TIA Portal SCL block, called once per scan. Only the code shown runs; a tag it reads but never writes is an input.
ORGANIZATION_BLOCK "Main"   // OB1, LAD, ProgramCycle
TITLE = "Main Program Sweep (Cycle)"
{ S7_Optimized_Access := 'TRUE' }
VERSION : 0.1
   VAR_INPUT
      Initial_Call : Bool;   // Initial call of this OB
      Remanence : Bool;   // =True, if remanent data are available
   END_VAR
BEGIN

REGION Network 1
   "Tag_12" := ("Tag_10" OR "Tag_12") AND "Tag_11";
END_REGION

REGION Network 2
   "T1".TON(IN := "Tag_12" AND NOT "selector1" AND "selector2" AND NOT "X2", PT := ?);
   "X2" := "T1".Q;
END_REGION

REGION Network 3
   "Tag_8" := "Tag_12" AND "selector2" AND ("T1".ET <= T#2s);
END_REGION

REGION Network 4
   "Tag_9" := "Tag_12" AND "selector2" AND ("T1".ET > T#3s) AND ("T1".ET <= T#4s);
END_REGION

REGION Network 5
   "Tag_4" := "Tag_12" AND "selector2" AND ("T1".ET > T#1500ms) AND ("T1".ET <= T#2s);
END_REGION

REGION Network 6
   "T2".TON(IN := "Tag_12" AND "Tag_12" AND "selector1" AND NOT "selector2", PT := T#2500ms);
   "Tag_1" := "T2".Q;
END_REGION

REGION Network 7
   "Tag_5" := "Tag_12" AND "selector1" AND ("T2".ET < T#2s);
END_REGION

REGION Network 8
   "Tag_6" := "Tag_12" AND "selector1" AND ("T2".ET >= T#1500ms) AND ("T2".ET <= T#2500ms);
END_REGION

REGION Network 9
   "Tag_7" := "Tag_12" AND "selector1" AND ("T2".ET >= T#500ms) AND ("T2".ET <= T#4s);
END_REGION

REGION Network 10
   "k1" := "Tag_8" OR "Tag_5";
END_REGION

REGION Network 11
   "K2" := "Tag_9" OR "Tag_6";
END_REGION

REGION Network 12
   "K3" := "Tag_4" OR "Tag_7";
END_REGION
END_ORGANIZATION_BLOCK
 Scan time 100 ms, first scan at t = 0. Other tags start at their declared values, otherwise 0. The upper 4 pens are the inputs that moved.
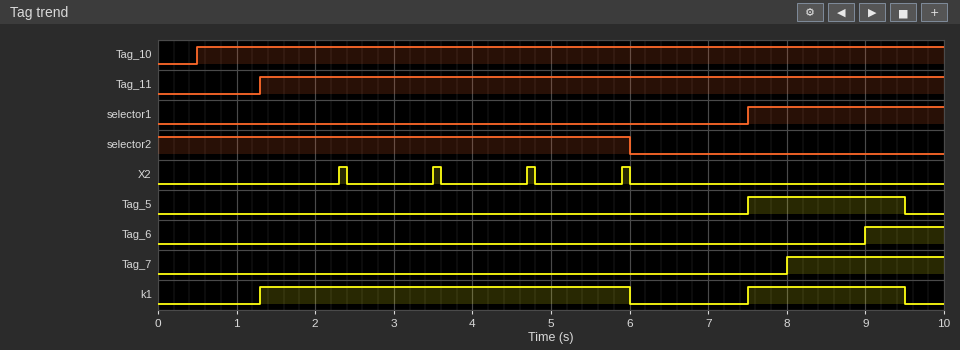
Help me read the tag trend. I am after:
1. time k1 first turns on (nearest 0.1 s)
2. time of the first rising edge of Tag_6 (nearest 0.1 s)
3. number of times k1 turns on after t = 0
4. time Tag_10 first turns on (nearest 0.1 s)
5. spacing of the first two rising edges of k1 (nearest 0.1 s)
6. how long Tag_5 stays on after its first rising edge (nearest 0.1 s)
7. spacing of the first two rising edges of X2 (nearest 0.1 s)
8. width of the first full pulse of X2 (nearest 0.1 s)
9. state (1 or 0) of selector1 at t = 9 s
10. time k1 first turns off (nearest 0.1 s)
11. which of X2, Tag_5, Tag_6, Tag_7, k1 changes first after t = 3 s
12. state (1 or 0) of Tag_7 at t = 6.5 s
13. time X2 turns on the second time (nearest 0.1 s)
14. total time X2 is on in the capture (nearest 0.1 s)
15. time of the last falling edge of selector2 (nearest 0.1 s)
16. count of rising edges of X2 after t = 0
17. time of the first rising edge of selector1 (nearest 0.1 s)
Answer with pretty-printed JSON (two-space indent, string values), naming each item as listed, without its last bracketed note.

{
  "time k1 first turns on": "1.3 s",
  "time of the first rising edge of Tag_6": "9.0 s",
  "number of times k1 turns on after t = 0": "2",
  "time Tag_10 first turns on": "0.5 s",
  "spacing of the first two rising edges of k1": "6.2 s",
  "how long Tag_5 stays on after its first rising edge": "2.0 s",
  "spacing of the first two rising edges of X2": "1.2 s",
  "width of the first full pulse of X2": "0.1 s",
  "state (1 or 0) of selector1 at t = 9 s": "1",
  "time k1 first turns off": "6.0 s",
  "which of X2, Tag_5, Tag_6, Tag_7, k1 changes first after t = 3 s": "X2",
  "state (1 or 0) of Tag_7 at t = 6.5 s": "0",
  "time X2 turns on the second time": "3.5 s",
  "total time X2 is on in the capture": "0.4 s",
  "time of the last falling edge of selector2": "6.0 s",
  "count of rising edges of X2 after t = 0": "4",
  "time of the first rising edge of selector1": "7.5 s"
}
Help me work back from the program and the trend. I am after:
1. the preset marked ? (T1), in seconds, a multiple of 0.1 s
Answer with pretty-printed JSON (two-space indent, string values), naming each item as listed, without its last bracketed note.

{
  "the preset marked ? (T1), in seconds, a multiple of 0.1 s": "1.0 s"
}
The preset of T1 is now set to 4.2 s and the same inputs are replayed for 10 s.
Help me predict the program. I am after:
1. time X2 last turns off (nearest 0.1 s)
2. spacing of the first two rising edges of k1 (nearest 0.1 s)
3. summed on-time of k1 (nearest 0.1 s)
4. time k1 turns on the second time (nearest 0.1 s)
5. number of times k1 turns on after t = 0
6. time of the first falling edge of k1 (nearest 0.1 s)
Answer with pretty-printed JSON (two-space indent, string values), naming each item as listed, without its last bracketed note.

{
  "time X2 last turns off": "5.6 s",
  "spacing of the first two rising edges of k1": "4.3 s",
  "summed on-time of k1": "4.5 s",
  "time k1 turns on the second time": "5.6 s",
  "number of times k1 turns on after t = 0": "3",
  "time of the first falling edge of k1": "3.4 s"
}
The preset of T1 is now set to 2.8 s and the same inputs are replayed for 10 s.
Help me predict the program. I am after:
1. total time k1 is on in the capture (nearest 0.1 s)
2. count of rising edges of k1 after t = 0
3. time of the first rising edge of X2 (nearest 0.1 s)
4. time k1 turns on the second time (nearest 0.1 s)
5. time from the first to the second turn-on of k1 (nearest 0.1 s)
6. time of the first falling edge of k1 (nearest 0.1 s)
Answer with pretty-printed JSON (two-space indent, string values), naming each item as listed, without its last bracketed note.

{
  "total time k1 is on in the capture": "5.9 s",
  "count of rising edges of k1 after t = 0": "3",
  "time of the first rising edge of X2": "4.1 s",
  "time k1 turns on the second time": "4.2 s",
  "time from the first to the second turn-on of k1": "2.9 s",
  "time of the first falling edge of k1": "3.4 s"
}
